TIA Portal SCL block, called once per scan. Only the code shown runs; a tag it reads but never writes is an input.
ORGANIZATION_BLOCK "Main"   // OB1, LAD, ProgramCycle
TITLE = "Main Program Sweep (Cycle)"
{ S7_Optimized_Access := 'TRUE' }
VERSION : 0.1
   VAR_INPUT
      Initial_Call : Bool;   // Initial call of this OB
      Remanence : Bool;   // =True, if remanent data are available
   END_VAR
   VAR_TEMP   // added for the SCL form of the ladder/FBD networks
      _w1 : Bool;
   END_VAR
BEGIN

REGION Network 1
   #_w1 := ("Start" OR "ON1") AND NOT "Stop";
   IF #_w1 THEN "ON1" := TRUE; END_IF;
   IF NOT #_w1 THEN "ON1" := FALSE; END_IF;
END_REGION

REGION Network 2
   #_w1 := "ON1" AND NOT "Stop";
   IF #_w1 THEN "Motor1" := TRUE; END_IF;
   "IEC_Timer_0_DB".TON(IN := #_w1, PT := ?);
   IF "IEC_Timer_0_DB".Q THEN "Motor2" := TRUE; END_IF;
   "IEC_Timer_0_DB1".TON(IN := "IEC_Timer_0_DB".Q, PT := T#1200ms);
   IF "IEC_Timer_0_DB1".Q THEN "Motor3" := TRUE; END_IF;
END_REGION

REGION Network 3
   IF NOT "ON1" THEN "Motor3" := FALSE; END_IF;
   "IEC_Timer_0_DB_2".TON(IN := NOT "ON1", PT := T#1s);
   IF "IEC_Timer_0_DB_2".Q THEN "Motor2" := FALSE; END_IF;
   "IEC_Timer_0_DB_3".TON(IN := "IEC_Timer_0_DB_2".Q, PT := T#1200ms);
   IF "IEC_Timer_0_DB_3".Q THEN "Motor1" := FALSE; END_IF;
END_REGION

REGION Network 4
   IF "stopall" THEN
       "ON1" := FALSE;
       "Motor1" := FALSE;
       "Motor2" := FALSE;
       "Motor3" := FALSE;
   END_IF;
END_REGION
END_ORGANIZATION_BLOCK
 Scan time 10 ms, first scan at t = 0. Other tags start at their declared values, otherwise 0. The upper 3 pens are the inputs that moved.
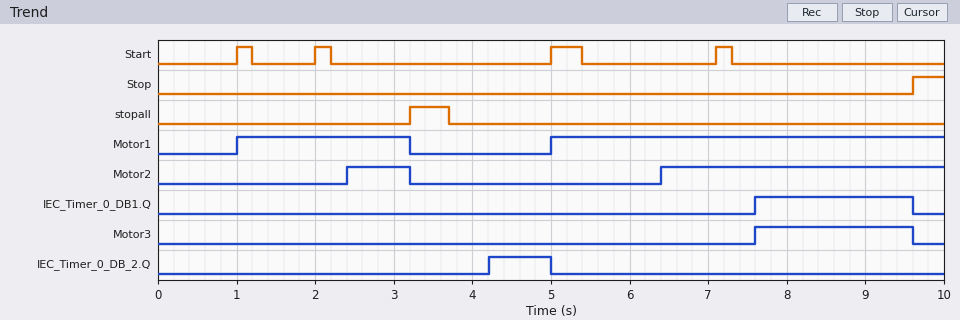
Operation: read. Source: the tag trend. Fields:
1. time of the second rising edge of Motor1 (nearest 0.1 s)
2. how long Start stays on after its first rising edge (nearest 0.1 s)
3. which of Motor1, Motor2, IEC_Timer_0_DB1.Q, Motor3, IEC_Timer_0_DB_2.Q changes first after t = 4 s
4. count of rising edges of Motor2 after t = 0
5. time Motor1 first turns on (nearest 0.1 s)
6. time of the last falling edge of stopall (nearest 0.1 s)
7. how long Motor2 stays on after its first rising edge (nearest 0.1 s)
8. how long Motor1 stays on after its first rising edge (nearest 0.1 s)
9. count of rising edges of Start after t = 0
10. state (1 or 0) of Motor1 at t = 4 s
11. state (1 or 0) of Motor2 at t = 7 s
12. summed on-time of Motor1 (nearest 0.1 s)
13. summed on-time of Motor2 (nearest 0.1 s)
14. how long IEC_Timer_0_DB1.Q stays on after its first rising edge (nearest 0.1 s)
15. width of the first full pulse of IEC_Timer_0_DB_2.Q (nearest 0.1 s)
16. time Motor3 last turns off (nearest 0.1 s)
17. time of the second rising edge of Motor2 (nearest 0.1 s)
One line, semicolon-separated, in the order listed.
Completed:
5.0 s; 0.2 s; IEC_Timer_0_DB_2.Q; 2; 1.0 s; 3.7 s; 0.8 s; 2.2 s; 4; 0; 1; 7.2 s; 4.4 s; 2.0 s; 0.8 s; 9.6 s; 6.4 s
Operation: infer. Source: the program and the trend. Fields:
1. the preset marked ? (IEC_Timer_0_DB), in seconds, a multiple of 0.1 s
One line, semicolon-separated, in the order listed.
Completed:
1.4 s
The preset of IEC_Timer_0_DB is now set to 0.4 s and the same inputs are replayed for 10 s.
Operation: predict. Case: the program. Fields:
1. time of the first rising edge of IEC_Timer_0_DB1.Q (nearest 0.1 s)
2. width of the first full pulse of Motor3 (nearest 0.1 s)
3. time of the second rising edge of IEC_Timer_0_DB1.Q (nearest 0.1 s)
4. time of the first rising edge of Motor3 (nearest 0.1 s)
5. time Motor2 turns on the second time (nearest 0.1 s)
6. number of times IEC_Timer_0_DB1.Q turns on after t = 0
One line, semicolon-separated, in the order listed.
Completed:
2.6 s; 0.6 s; 6.6 s; 2.6 s; 5.4 s; 2
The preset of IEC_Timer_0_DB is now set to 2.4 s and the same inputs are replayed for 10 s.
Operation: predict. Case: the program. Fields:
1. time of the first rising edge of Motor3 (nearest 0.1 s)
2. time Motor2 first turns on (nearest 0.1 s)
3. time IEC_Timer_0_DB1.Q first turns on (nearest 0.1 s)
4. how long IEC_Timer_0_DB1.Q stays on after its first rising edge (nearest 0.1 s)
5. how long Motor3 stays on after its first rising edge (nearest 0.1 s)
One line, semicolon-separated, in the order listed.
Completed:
8.6 s; 7.4 s; 8.6 s; 1.0 s; 1.0 s
